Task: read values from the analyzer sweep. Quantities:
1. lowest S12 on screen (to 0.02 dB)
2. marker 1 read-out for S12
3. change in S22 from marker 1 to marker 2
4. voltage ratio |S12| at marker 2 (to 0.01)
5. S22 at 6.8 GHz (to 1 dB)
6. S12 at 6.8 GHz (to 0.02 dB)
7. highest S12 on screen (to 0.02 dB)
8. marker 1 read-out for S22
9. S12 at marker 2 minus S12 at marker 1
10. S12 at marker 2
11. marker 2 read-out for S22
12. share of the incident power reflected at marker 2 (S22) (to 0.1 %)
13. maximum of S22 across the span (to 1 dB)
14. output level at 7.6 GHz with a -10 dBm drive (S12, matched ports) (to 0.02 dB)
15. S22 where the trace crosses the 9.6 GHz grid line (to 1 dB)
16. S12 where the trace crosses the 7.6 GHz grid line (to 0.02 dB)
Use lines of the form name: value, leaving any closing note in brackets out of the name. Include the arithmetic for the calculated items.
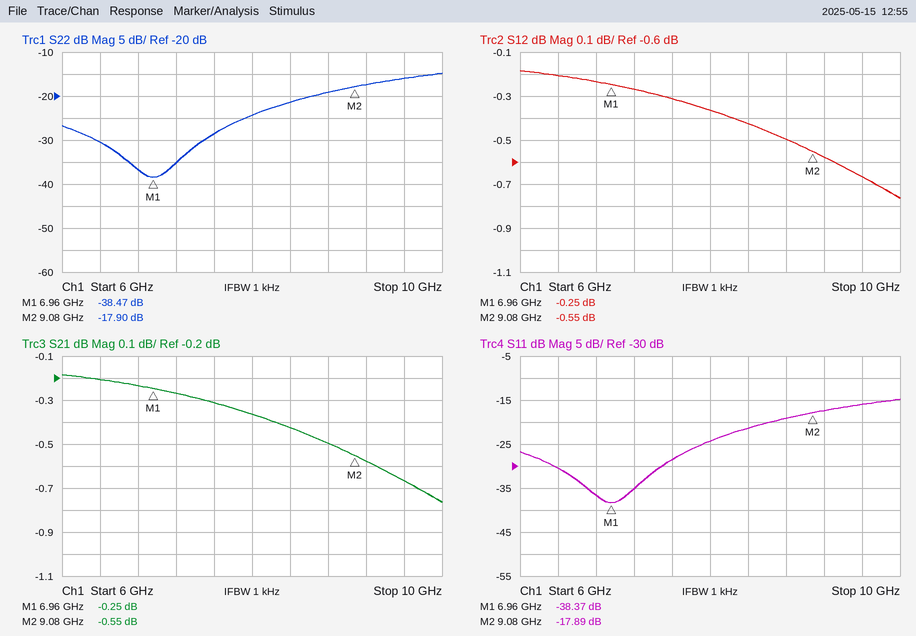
lowest S12 on screen: -0.76 dB
marker 1 read-out for S12: -0.25 dB
change in S22 from marker 1 to marker 2: -17.9 − (-38.47) = 20.57 dB
voltage ratio |S12| at marker 2: 10^(-0.55/20) ≈ 0.94
S22 at 6.8 GHz: -37 dB
S12 at 6.8 GHz: -0.24 dB
highest S12 on screen: -0.18 dB
marker 1 read-out for S22: -38.47 dB
S12 at marker 2 minus S12 at marker 1: -0.55 − (-0.25) = -0.30 dB
S12 at marker 2: -0.55 dB
marker 2 read-out for S22: -17.90 dB
share of the incident power reflected at marker 2 (S22): 10^(-17.9/10) ≈ 1.6 %
maximum of S22 across the span: -15 dB
output level at 7.6 GHz with a -10 dBm drive (S12, matched ports): -10 dBm + (-0.32 dB) = -10.32 dBm
S22 where the trace crosses the 9.6 GHz grid line: -16 dB
S12 where the trace crosses the 7.6 GHz grid line: -0.32 dB
